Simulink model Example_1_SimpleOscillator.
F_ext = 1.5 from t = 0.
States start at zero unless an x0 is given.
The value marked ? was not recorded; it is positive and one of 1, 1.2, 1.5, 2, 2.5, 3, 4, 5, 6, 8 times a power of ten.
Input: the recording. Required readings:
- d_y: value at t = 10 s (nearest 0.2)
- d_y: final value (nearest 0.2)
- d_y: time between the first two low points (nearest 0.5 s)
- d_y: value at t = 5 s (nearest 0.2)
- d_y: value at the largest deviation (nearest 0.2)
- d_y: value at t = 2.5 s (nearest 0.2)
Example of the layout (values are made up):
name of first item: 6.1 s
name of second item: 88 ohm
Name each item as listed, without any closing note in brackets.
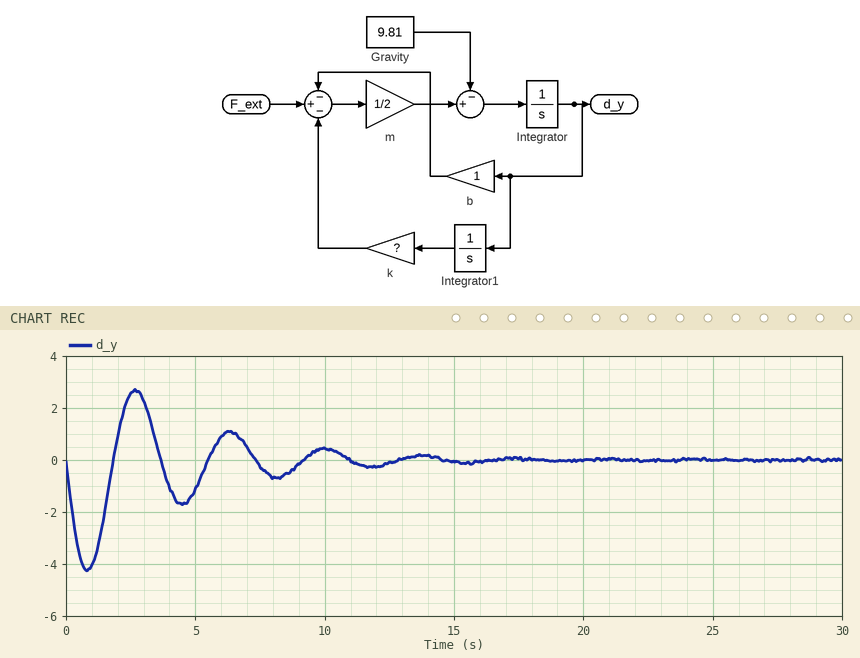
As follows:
d_y: value at t = 10 s: 0.4
d_y: final value: 0.0
d_y: time between the first two low points: 3.5 s
d_y: value at t = 5 s: -1.2
d_y: value at the largest deviation: -4.2
d_y: value at t = 2.5 s: 2.6
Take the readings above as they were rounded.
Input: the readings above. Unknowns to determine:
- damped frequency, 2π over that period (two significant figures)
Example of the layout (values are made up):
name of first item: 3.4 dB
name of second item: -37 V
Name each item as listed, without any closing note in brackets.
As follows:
damped frequency, 2π over that period: 1.8 rad/s
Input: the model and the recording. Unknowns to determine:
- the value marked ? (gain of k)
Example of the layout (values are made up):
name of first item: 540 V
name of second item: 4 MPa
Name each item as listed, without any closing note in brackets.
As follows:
the value marked ?: 6
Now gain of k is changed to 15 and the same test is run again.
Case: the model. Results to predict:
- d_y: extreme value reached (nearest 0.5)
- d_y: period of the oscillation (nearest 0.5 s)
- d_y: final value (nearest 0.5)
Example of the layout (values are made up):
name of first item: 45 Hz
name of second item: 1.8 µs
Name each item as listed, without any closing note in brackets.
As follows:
d_y: extreme value reached: -3.0
d_y: period of the oscillation: 2.5 s
d_y: final value: 0.0
